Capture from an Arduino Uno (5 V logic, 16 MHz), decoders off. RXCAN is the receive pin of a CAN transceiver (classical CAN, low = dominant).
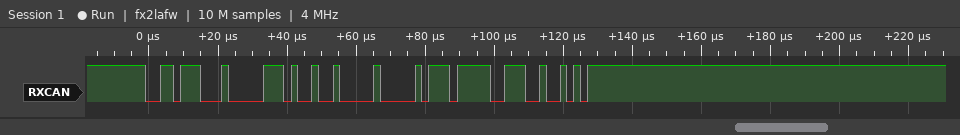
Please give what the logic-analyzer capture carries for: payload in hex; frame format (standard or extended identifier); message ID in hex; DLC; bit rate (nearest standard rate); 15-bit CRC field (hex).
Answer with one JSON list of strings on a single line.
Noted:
["49 00 1D", "standard", "0x371", "3", "500 kbit/s", "0x7B92"]
